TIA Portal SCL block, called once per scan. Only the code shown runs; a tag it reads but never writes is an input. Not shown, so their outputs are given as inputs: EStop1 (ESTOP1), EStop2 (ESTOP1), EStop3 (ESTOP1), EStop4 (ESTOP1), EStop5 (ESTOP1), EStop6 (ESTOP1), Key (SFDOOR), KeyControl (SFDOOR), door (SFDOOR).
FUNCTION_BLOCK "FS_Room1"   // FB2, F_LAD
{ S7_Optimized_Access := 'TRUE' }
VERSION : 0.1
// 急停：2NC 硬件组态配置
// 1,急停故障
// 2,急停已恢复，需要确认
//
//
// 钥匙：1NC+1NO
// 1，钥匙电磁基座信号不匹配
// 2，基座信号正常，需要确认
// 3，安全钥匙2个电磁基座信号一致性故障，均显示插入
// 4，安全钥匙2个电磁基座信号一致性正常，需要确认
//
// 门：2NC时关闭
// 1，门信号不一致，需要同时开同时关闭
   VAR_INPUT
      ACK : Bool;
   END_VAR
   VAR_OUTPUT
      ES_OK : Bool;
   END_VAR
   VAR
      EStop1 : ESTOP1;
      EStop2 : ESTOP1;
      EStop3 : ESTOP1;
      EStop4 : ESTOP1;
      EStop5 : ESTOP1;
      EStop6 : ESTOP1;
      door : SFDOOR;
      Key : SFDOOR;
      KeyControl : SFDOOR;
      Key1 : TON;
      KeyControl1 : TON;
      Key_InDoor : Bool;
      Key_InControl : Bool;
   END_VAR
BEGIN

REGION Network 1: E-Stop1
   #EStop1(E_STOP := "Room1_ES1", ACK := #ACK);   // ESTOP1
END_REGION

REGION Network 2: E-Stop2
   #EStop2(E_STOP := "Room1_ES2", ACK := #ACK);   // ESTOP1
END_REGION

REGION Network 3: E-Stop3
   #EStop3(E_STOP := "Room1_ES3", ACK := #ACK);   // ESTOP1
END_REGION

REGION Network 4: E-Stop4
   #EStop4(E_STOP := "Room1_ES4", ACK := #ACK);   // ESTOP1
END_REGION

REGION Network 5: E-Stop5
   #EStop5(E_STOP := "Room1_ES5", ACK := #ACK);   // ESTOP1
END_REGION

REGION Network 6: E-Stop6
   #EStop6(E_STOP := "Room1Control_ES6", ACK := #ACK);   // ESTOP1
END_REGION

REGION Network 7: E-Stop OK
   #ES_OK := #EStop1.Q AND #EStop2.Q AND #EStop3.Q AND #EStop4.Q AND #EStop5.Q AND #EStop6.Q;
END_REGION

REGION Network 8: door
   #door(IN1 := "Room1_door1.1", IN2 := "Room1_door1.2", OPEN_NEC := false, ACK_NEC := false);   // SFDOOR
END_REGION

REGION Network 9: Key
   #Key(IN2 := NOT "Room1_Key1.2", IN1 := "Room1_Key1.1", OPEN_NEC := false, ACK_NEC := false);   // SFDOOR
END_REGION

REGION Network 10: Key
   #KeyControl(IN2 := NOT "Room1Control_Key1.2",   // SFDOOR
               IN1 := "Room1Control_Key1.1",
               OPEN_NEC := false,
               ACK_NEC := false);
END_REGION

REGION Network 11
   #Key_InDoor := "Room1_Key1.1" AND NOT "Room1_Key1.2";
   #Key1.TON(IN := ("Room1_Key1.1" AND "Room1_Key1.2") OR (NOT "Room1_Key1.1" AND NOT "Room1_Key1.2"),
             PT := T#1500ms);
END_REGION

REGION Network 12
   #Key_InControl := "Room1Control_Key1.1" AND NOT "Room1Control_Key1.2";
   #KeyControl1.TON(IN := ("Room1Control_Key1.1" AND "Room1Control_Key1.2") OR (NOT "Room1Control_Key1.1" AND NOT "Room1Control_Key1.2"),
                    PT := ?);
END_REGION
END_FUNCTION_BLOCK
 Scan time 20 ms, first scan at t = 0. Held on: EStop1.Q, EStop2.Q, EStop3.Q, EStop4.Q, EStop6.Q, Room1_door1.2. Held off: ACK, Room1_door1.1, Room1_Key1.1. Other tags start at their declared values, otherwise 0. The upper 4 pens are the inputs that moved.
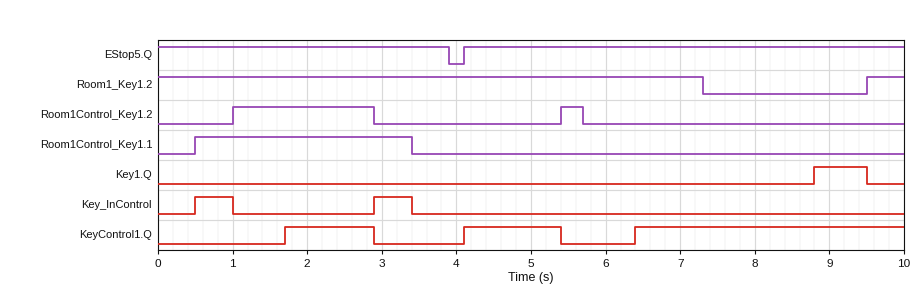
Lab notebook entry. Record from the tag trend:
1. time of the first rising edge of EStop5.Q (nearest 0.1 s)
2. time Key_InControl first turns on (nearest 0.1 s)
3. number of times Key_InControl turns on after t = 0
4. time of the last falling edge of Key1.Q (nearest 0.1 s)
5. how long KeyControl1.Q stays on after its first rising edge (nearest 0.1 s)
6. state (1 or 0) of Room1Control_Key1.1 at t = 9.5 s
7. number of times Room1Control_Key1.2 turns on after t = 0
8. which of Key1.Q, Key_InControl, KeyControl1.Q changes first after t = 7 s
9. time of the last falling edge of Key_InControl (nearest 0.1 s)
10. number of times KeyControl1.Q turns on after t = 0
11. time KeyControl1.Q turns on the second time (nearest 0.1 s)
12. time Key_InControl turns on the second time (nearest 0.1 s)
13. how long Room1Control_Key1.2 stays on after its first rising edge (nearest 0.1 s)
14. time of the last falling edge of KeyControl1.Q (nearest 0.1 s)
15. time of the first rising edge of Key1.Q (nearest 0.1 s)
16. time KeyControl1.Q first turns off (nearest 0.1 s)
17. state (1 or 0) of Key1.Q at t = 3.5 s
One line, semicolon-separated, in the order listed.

4.1 s; 0.5 s; 2; 9.5 s; 1.2 s; 0; 2; Key1.Q; 3.4 s; 3; 4.1 s; 2.9 s; 1.9 s; 5.4 s; 8.8 s; 2.9 s; 0
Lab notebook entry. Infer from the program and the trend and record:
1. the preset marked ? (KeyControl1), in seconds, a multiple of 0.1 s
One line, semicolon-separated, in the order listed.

0.7 s
